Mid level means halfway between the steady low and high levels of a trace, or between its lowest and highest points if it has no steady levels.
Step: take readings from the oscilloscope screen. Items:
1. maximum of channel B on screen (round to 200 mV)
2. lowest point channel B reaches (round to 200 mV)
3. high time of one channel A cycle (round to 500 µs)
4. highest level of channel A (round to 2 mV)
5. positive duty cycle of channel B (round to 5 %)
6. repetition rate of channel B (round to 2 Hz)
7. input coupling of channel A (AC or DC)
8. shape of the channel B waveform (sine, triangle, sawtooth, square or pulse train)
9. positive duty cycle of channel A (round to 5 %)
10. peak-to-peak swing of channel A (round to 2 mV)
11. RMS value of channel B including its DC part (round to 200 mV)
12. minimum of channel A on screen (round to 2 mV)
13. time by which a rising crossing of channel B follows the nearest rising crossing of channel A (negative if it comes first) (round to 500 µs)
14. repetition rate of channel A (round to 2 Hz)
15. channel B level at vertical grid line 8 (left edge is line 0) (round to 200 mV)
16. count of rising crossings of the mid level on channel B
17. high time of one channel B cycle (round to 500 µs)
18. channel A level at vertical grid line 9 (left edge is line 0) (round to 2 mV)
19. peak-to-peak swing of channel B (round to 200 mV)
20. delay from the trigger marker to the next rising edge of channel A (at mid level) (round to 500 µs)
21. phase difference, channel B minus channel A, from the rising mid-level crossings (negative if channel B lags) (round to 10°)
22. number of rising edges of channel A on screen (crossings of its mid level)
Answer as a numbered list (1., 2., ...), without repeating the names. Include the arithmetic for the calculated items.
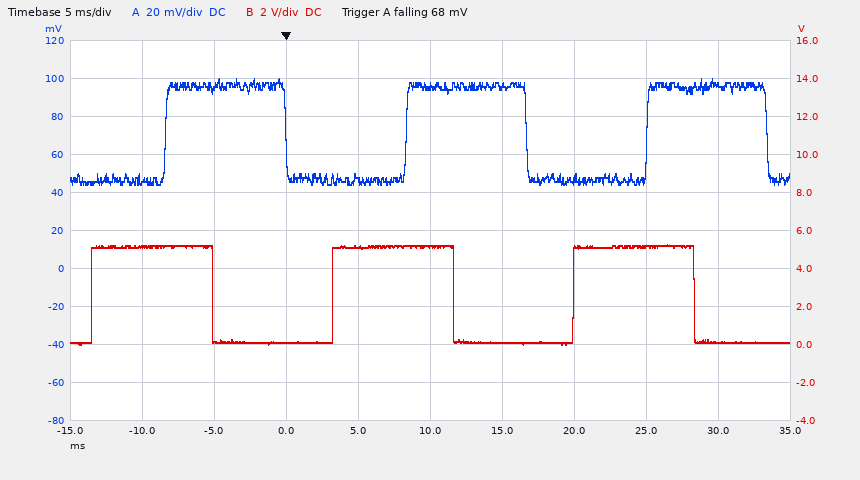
1. 5.2 V
2. 0.0 V
3. 8.5 ms
4. 100 mV
5. 50 %
6. 60 Hz
7. DC
8. square
9. 50 %
10. 100 mV − (44 mV) = 56 mV
11. √(0.5 × (5.2 V)² + 0.5 × (0.0 V)²) ≈ 3.68 V, so 3.6 V to the nearest 200 mV
12. 44 mV
13. -5.0 ms
14. 60 Hz
15. 5.2 V
16. 3
17. 8.5 ms
18. 96 mV
19. 5.2 V − (0.0 V) = 5.2 V
20. 8.5 ms
21. +110°
22. 3
